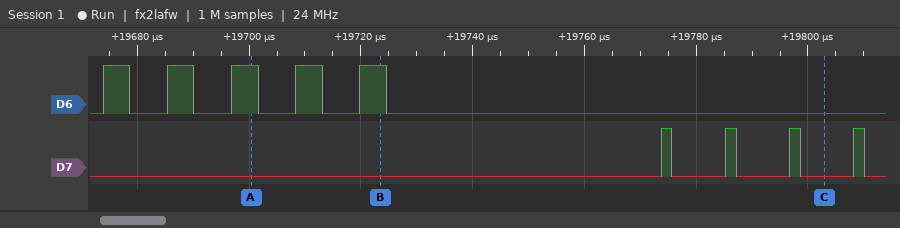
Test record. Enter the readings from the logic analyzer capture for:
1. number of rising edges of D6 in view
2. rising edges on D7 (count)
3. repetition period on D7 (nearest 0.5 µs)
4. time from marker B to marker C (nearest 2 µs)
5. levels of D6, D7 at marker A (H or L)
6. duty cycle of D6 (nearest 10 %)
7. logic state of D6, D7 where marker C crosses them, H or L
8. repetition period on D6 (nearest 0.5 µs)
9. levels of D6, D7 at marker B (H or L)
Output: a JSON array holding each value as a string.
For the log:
["5", "4", "11.5 µs", "80 µs", "D6=H, D7=L", "40 %", "D6=L, D7=L", "11.5 µs", "D6=H, D7=L"]
